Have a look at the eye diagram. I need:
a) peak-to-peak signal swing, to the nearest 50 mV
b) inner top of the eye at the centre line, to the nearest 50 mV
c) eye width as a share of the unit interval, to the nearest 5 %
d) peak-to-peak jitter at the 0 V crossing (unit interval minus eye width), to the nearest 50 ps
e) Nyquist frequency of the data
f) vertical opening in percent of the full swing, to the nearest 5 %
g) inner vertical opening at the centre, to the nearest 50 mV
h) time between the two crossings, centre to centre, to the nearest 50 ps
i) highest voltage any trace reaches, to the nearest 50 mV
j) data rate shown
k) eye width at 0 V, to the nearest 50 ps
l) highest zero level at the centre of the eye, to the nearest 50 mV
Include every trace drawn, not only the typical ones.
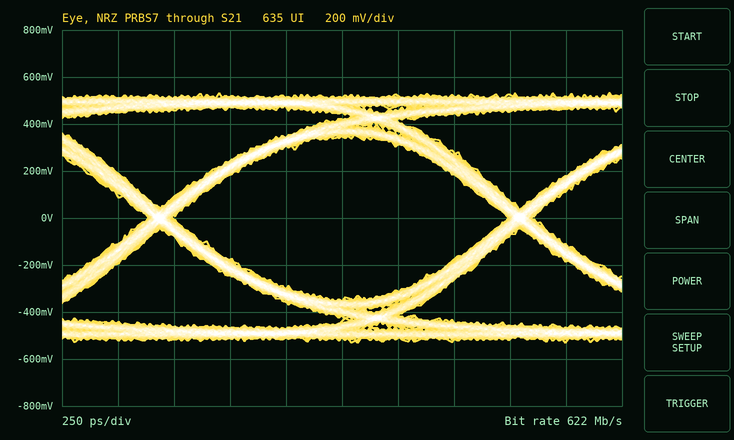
1.05 V
350 mV
95 %
100 ps
311 MHz
65 %
700 mV
1.60 ns
550 mV
622 Mb/s
1.50 ns
-350 mV
